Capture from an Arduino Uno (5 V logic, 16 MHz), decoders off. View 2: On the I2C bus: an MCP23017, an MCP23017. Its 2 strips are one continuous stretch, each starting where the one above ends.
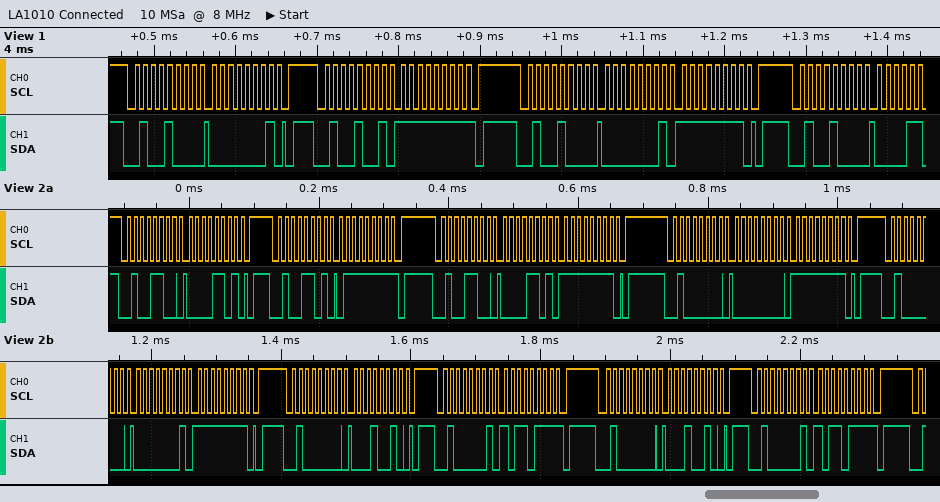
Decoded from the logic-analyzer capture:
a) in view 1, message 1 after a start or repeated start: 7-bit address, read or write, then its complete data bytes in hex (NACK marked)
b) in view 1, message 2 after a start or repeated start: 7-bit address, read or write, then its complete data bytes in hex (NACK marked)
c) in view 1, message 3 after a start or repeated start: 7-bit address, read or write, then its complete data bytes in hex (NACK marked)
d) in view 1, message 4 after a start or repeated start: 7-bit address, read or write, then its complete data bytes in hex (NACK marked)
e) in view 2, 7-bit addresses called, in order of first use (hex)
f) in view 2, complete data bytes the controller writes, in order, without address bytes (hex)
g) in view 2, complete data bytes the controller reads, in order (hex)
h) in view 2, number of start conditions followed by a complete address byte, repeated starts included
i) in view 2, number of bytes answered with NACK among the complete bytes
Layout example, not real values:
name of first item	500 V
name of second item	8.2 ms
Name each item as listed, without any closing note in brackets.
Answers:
in view 1, message 1 after a start or repeated start: 7-bit address, read or write, then its complete data bytes in hex	0x24 write: 01
in view 1, message 2 after a start or repeated start: 7-bit address, read or write, then its complete data bytes in hex	0x24 read: FF NACK
in view 1, message 3 after a start or repeated start: 7-bit address, read or write, then its complete data bytes in hex	0x24 write: 01 FF
in view 1, message 4 after a start or repeated start: 7-bit address, read or write, then its complete data bytes in hex	0x24 write
in view 2, 7-bit addresses called, in order of first use	0x26 0x20
in view 2, complete data bytes the controller writes, in order, without address bytes	0D 0D FF 00 FF 01 FF 12 12
in view 2, complete data bytes the controller reads, in order	7F B7 B7
in view 2, number of start conditions followed by a complete address byte, repeated starts included	9
in view 2, number of bytes answered with NACK among the complete bytes	3
